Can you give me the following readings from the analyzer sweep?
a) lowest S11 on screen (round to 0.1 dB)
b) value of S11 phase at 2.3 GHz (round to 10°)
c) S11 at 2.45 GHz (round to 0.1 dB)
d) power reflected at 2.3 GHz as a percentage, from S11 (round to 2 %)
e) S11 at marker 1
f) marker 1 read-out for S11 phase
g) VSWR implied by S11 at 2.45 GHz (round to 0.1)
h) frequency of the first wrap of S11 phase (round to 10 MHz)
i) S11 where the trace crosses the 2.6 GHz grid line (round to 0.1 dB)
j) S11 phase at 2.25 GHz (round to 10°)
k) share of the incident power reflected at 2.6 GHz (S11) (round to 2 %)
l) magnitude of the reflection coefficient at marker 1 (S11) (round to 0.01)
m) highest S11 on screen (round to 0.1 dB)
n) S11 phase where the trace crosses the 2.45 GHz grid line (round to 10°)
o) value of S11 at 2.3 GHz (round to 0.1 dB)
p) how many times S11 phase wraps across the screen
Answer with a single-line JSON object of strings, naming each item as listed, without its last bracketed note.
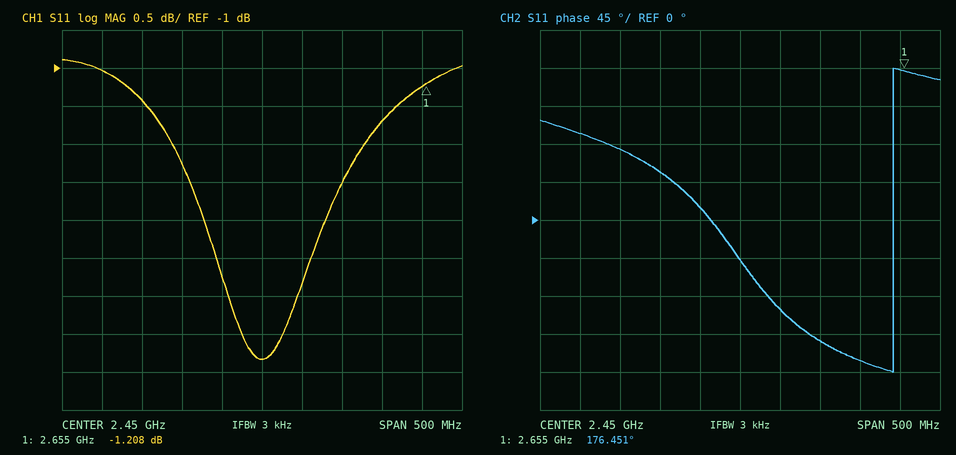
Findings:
{"lowest S11 on screen": "-4.8 dB", "value of S11 phase at 2.3 GHz": "80°", "S11 at 2.45 GHz": "-4.8 dB", "power reflected at 2.3 GHz as a percentage, from S11": "72 %", "S11 at marker 1": "-1.208 dB", "marker 1 read-out for S11 phase": "176.451°", "VSWR implied by S11 at 2.45 GHz": "3.7", "frequency of the first wrap of S11 phase": "2.64 GHz", "S11 where the trace crosses the 2.6 GHz grid line": "-1.7 dB", "S11 phase at 2.25 GHz": "100°", "share of the incident power reflected at 2.6 GHz (S11)": "68 %", "magnitude of the reflection coefficient at marker 1 (S11)": "0.87", "highest S11 on screen": "-0.9 dB", "S11 phase where the trace crosses the 2.45 GHz grid line": "-50°", "value of S11 at 2.3 GHz": "-1.4 dB", "how many times S11 phase wraps across the screen": "1"}
